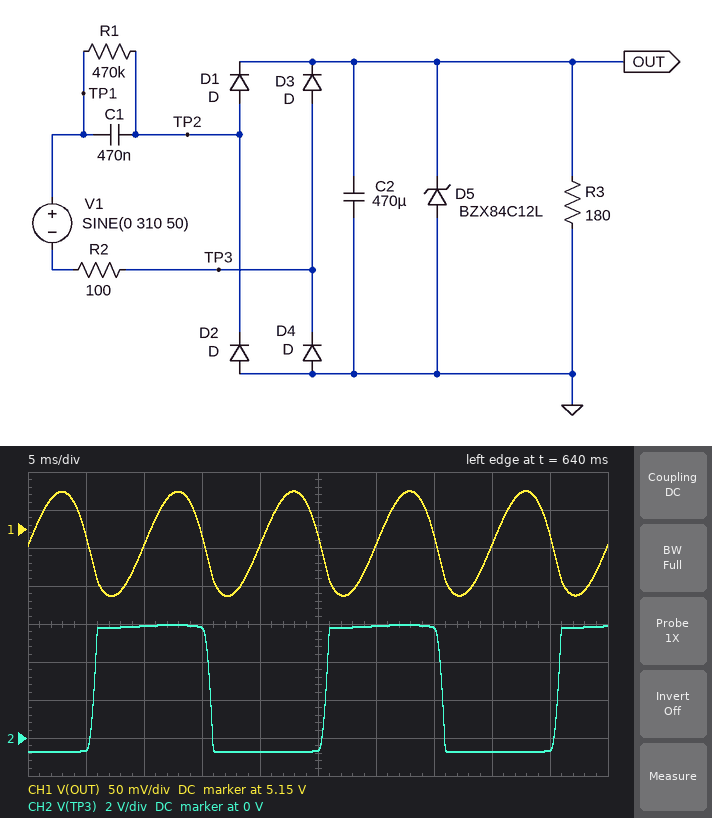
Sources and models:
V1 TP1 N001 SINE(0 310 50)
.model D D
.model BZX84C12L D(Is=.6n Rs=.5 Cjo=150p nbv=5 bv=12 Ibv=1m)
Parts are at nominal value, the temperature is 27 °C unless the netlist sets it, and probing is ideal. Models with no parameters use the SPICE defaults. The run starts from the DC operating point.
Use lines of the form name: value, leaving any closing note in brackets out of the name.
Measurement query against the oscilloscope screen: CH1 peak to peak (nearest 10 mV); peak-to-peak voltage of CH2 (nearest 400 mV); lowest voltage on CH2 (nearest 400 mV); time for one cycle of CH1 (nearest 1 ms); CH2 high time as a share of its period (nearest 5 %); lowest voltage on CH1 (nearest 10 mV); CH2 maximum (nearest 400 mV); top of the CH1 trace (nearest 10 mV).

CH1 peak to peak: 140 mV
peak-to-peak voltage of CH2: 6.8 V
lowest voltage on CH2: -800 mV
time for one cycle of CH1: 10 ms
CH2 high time as a share of its period: 50 %
lowest voltage on CH1: 5.06 V
CH2 maximum: 6.0 V
top of the CH1 trace: 5.20 V
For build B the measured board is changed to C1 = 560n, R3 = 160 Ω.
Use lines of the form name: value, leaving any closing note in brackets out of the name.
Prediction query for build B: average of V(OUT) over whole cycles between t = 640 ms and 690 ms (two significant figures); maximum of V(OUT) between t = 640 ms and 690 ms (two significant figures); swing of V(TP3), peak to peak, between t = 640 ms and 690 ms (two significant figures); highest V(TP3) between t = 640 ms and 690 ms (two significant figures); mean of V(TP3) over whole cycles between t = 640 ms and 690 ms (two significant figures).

average of V(OUT) over whole cycles between t = 640 ms and 690 ms: 5.4 V
maximum of V(OUT) between t = 640 ms and 690 ms: 5.5 V
swing of V(TP3), peak to peak, between t = 640 ms and 690 ms: 7.0 V
highest V(TP3) between t = 640 ms and 690 ms: 6.3 V
mean of V(TP3) over whole cycles between t = 640 ms and 690 ms: 2.7 V
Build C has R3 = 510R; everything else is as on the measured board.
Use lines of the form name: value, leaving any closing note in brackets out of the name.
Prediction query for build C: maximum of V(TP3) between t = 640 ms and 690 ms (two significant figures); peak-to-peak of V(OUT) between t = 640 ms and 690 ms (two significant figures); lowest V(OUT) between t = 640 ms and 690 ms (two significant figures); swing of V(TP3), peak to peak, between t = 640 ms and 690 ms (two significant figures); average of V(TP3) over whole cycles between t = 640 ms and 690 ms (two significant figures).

maximum of V(TP3) between t = 640 ms and 690 ms: 13 V
peak-to-peak of V(OUT) between t = 640 ms and 690 ms: 150 mV
lowest V(OUT) between t = 640 ms and 690 ms: 12 V
swing of V(TP3), peak to peak, between t = 640 ms and 690 ms: 14 V
average of V(TP3) over whole cycles between t = 640 ms and 690 ms: 6.1 V
